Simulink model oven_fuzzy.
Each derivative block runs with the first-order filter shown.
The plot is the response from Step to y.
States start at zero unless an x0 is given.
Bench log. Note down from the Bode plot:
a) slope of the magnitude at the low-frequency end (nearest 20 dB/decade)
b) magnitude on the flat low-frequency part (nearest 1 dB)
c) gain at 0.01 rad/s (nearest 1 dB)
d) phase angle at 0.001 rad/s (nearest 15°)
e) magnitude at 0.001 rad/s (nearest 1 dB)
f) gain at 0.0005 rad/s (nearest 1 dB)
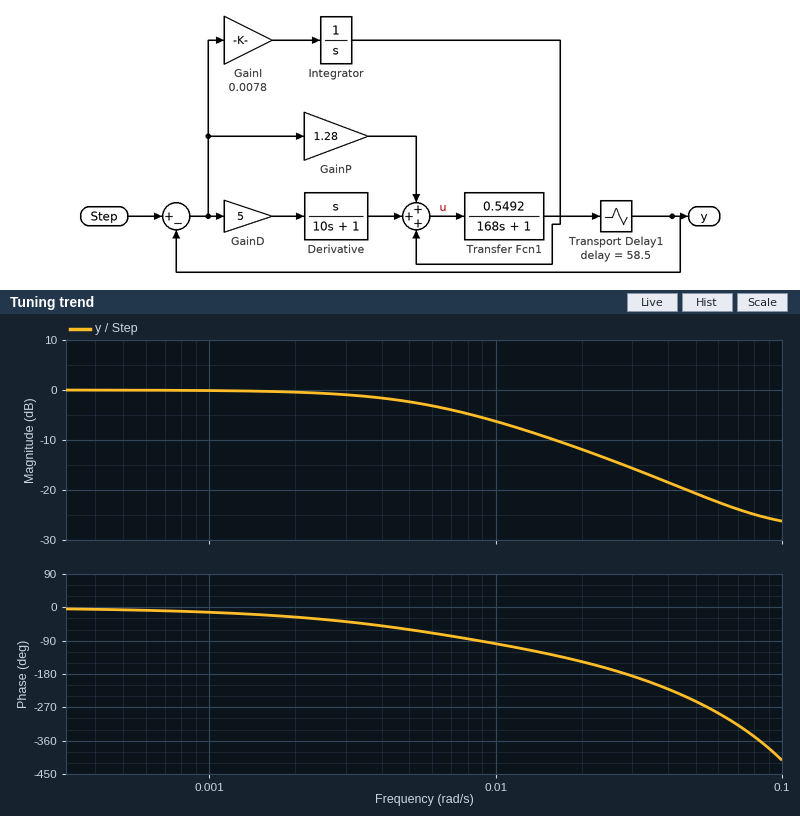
0 dB/decade
0 dB
-6 dB
-15°
0 dB
0 dB
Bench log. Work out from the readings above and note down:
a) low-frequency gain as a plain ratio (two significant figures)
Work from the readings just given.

1.0
